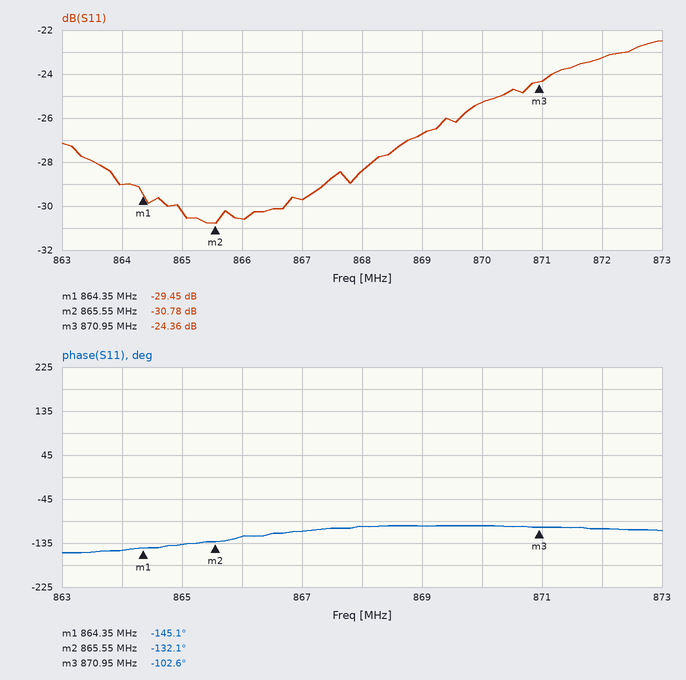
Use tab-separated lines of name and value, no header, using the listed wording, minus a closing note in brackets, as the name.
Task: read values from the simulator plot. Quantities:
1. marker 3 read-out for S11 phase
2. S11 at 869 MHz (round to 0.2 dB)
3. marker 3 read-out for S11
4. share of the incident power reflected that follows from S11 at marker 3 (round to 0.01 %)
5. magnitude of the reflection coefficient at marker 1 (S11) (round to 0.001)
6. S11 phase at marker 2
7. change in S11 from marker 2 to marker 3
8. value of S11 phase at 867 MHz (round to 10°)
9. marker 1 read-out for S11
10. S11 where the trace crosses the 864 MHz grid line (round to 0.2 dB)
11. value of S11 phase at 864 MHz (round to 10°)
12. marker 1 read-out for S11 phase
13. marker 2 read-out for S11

marker 3 read-out for S11 phase	-102.6°
S11 at 869 MHz	-26.8 dB
marker 3 read-out for S11	-24.36 dB
share of the incident power reflected that follows from S11 at marker 3	0.37 %
magnitude of the reflection coefficient at marker 1 (S11)	0.034
S11 phase at marker 2	-132.1°
change in S11 from marker 2 to marker 3	6.42 dB
value of S11 phase at 867 MHz	-110°
marker 1 read-out for S11	-29.45 dB
S11 where the trace crosses the 864 MHz grid line	-29.0 dB
value of S11 phase at 864 MHz	-150°
marker 1 read-out for S11 phase	-145.1°
marker 2 read-out for S11	-30.78 dB
